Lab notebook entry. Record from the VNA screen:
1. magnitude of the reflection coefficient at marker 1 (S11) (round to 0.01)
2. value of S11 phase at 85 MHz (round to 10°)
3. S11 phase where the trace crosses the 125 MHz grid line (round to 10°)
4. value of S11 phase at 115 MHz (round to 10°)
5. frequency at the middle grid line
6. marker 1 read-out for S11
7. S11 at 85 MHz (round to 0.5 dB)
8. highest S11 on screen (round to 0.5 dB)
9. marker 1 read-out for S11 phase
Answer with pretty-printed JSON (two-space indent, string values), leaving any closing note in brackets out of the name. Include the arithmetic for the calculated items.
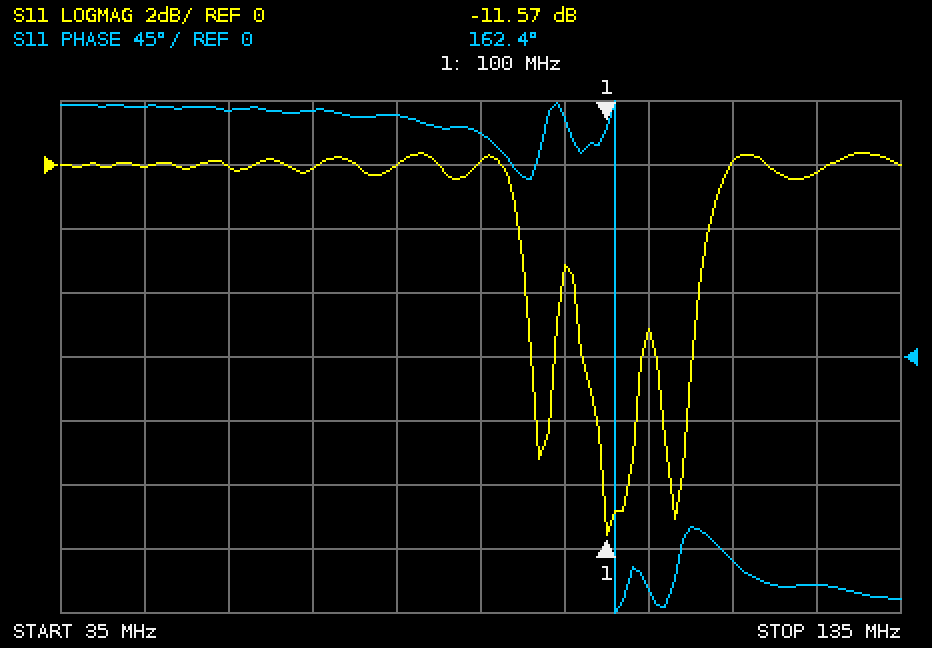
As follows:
{
  "magnitude of the reflection coefficient at marker 1 (S11)": "10^(-11.57/20) ≈ 0.26",
  "value of S11 phase at 85 MHz": "160°",
  "S11 phase where the trace crosses the 125 MHz grid line": "-160°",
  "value of S11 phase at 115 MHz": "-140°",
  "frequency at the middle grid line": "85 MHz",
  "marker 1 read-out for S11": "-11.57 dB",
  "S11 at 85 MHz": "0.0 dB",
  "highest S11 on screen": "0.5 dB",
  "marker 1 read-out for S11 phase": "162.4°"
}
